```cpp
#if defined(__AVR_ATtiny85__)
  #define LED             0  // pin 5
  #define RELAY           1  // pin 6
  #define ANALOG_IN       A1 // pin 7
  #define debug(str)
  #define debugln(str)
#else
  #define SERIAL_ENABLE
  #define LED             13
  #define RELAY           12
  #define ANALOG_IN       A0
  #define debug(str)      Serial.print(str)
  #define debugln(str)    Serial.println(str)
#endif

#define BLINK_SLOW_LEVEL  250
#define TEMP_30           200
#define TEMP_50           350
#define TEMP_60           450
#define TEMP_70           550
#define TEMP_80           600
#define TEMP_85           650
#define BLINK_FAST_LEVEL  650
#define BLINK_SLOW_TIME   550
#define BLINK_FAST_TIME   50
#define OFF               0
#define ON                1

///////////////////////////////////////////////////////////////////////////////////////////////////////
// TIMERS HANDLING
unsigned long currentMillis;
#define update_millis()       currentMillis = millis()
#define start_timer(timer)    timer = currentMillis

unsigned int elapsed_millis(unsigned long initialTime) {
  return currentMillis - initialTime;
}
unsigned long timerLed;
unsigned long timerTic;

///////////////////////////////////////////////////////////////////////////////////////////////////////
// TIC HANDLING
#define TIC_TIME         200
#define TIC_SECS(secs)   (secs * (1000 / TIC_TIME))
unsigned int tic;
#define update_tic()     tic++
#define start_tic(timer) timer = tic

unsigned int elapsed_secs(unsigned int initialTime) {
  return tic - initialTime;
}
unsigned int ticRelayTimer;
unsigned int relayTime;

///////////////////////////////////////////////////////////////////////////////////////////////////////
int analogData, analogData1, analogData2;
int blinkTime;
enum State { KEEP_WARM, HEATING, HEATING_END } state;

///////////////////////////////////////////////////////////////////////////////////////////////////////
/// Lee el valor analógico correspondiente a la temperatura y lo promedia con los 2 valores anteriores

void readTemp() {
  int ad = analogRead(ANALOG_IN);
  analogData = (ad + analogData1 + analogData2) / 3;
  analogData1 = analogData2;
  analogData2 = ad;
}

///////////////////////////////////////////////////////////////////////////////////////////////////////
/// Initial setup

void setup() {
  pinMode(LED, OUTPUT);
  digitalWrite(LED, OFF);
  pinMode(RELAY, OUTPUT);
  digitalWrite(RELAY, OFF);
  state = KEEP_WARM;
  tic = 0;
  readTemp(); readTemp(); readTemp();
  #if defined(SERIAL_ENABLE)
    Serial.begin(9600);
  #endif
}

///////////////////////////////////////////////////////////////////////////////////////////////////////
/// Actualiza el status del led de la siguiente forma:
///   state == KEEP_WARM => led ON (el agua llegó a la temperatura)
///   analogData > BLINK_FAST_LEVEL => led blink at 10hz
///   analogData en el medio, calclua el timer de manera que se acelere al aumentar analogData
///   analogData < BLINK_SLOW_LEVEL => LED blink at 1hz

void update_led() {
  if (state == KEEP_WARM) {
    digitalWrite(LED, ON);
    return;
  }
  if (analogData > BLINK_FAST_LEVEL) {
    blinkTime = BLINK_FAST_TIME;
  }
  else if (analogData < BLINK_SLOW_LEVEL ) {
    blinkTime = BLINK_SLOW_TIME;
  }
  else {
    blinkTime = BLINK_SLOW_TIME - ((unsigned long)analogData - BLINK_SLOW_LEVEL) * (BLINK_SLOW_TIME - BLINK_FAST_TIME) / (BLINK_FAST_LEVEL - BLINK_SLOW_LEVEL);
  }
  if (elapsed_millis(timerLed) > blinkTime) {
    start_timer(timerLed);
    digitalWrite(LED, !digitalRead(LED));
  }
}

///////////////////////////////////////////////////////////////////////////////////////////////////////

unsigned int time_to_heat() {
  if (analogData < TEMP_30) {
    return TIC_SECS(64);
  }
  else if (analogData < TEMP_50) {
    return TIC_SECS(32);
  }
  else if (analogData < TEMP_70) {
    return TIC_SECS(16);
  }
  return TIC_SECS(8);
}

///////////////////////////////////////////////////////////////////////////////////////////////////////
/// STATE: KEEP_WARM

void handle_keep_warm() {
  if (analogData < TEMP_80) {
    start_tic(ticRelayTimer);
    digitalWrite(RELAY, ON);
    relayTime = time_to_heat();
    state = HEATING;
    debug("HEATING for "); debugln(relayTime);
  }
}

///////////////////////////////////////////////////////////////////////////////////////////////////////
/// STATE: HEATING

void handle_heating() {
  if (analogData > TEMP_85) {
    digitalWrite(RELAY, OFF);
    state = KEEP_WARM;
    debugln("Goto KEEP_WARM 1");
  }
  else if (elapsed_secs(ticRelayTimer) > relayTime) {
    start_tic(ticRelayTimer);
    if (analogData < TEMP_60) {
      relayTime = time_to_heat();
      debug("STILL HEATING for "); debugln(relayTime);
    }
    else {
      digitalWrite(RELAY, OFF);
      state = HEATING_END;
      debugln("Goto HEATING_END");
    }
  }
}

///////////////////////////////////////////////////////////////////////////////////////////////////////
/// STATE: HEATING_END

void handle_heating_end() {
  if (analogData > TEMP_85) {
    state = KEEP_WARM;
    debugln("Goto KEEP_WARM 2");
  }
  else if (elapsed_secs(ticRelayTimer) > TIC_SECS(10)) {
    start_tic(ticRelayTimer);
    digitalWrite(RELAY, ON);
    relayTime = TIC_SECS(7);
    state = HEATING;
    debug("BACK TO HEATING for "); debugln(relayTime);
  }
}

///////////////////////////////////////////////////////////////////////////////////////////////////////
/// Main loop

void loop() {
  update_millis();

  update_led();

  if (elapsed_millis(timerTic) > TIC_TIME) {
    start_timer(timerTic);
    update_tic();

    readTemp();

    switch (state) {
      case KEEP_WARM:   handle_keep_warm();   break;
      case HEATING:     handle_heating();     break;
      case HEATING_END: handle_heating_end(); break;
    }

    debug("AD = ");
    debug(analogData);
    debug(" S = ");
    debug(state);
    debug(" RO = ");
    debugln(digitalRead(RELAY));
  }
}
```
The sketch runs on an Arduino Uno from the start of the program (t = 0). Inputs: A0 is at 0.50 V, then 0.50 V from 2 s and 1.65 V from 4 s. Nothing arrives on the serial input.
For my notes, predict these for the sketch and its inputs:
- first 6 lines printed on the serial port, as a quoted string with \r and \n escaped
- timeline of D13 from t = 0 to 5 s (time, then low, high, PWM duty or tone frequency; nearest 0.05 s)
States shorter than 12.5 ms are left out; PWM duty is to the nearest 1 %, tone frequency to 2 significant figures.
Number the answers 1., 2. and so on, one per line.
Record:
1. "HEATING for 320\r\nAD = 102 S = 1 RO = 1\r\nAD = 102 S = 1 RO = 1\r\nAD = 102 S = 1 RO = 1\r\nAD = 102 S = 1 RO = 1\r\nAD = 102 S = 1 RO = 1\r\n"
2. 0 s high; 0.55 s low; 1.1 s high; 1.65 s low; 2.2 s high; 2.75 s low; 3.3 s high; 3.85 s low; 4.4 s high; 4.85 s low
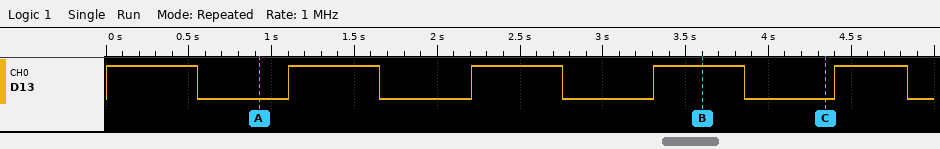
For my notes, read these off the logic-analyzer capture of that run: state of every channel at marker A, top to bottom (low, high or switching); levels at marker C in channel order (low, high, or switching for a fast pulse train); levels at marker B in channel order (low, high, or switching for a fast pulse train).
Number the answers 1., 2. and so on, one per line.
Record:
1. D13 low
2. D13 low
3. D13 high
